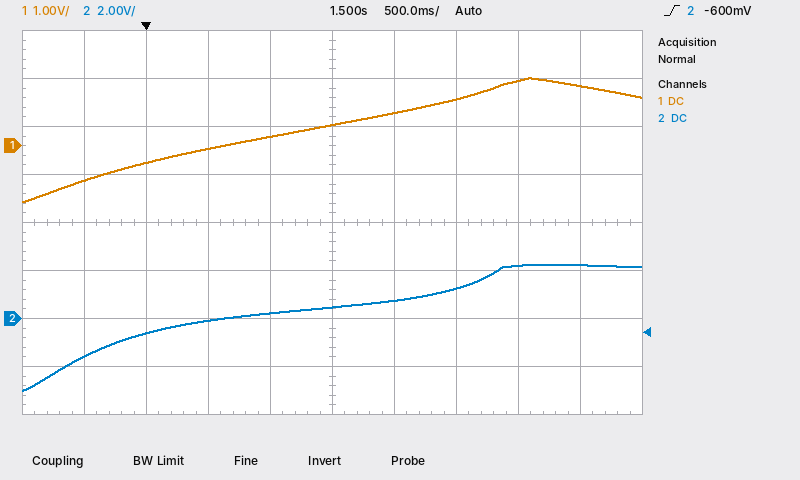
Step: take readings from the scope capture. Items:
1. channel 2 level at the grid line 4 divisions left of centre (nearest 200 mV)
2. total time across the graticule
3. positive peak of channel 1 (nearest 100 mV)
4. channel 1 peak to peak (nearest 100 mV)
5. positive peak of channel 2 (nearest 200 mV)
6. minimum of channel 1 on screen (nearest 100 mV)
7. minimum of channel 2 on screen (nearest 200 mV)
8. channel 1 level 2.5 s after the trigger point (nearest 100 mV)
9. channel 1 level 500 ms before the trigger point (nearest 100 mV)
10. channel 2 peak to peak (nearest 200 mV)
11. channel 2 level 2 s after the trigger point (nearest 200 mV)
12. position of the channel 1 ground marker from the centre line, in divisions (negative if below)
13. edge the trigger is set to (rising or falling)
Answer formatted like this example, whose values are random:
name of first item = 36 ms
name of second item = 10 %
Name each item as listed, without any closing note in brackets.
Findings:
channel 2 level at the grid line 4 divisions left of centre = -1.6 V
total time across the graticule = 5 s
positive peak of channel 1 = 1.4 V
channel 1 peak to peak = 2.6 V
positive peak of channel 2 = 2.2 V
minimum of channel 1 on screen = -1.2 V
minimum of channel 2 on screen = -3.0 V
channel 1 level 2.5 s after the trigger point = 1.0 V
channel 1 level 500 ms before the trigger point = -700 mV
channel 2 peak to peak = 5.2 V
channel 2 level 2 s after the trigger point = 800 mV
position of the channel 1 ground marker from the centre line, in divisions = +1.6 div
edge the trigger is set to = rising
